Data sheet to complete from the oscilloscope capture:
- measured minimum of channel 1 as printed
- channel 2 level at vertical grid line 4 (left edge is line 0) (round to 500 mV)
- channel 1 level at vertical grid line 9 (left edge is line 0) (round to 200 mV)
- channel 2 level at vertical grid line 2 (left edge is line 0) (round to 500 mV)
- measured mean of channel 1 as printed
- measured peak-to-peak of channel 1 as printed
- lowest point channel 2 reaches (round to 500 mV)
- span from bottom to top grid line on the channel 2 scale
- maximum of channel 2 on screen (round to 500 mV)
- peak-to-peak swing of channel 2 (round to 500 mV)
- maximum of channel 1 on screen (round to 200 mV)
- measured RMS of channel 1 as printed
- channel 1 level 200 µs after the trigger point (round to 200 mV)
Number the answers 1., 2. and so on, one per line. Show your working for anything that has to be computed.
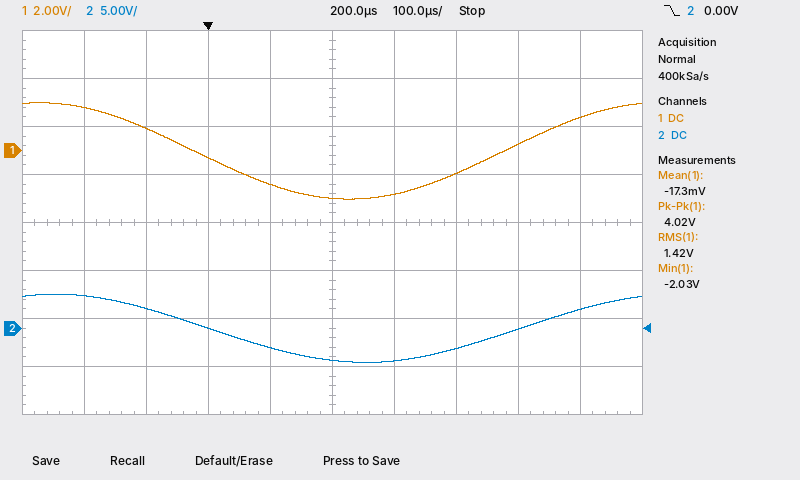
1. -2.03 V
2. -2.0 V
3. 1.4 V
4. 2.0 V
5. -17.3 mV
6. 4.02 V
7. -3.5 V
8. 40 V
9. 3.5 V
10. 3.5 V − (-3.5 V) = 7.0 V
11. 2.0 V
12. 1.42 V
13. -2.0 V
